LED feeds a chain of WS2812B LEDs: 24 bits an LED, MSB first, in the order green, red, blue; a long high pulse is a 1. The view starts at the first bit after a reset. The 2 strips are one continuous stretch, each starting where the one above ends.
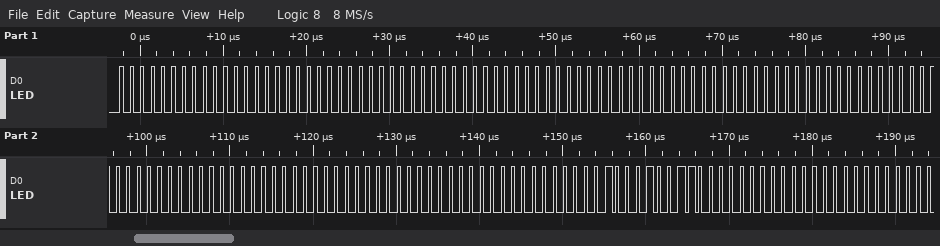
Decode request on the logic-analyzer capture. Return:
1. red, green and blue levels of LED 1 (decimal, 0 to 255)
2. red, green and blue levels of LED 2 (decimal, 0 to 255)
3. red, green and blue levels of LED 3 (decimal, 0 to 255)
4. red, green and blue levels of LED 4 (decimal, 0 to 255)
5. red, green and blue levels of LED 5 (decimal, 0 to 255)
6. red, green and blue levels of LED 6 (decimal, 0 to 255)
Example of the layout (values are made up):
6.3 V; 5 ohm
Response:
0, 0, 0; 0, 0, 0; 0, 0, 0; 0, 0, 0; 0, 0, 0; 38, 2, 0
